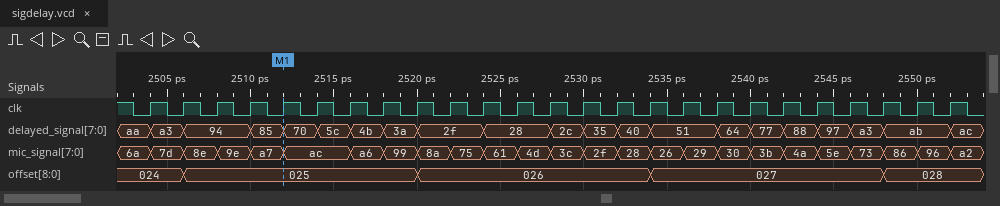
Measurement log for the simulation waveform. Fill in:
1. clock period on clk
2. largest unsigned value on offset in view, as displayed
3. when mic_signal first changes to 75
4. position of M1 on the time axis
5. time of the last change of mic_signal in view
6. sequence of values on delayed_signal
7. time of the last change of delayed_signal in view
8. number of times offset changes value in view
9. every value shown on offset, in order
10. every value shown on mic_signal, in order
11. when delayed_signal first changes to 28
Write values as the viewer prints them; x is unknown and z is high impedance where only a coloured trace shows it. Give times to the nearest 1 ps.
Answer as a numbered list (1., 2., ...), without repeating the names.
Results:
1. 2 ps
2. 028
3. 2522 ps
4. 2512 ps
5. 2552 ps
6. aa, a3, 94, 85, 70, 5c, 4b, 3a, 2f, 28, 2c, 35, 40, 51, 64, 77, 88, 97, a3, ab, ac
7. 2552 ps
8. 4
9. 024, 025, 026, 027, 028
10. 6a, 7d, 8e, 9e, a7, ac, a6, 99, 8a, 75, 61, 4d, 3c, 2f, 28, 26, 29, 30, 3b, 4a, 5e, 73, 86, 96, a2
11. 2524 ps
